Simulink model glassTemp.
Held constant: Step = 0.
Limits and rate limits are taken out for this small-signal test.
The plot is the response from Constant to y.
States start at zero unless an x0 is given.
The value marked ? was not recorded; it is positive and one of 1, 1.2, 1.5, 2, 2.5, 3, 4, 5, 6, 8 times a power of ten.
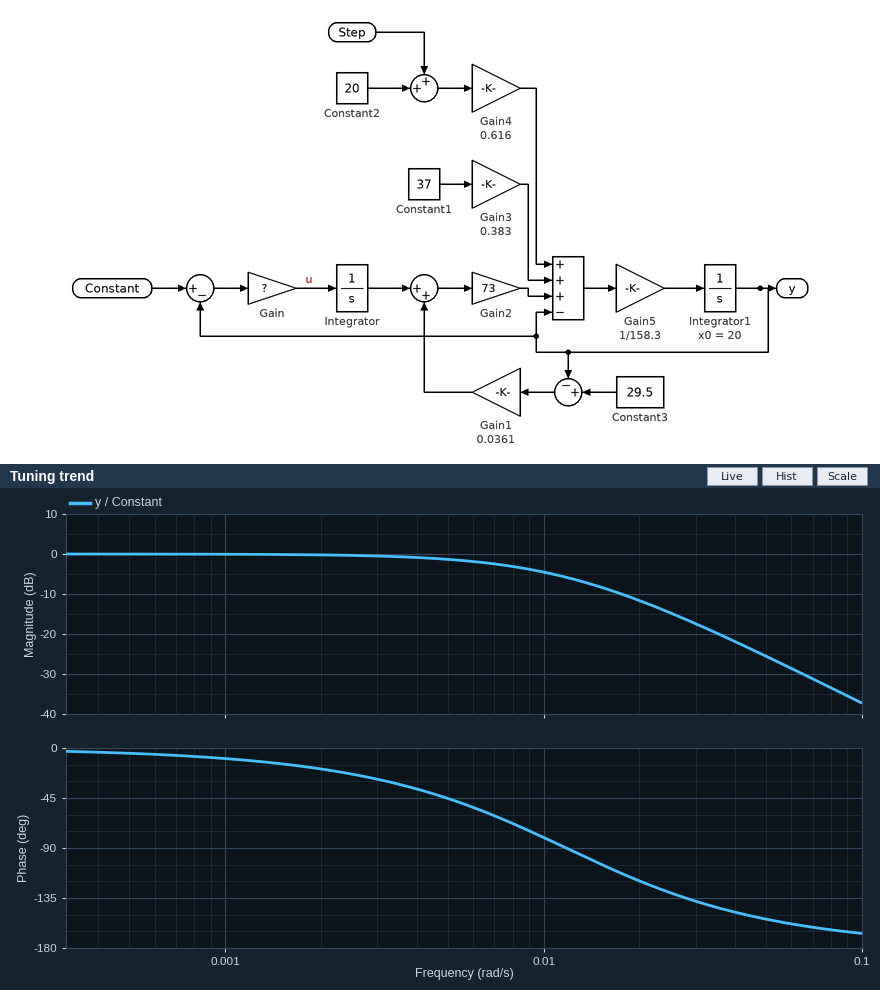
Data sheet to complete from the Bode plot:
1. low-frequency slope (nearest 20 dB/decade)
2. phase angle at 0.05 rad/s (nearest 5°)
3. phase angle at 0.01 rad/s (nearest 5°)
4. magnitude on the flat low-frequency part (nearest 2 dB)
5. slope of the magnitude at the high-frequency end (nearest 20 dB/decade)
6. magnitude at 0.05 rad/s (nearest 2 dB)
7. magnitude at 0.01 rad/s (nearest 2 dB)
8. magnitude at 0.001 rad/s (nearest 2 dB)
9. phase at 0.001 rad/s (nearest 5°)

0 dB/decade
-155°
-80°
0 dB
-40 dB/decade
-26 dB
-4 dB
0 dB
-10°
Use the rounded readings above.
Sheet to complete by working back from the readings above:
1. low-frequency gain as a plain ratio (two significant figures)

1.0
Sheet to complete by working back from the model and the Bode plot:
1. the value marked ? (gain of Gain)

0.0003
